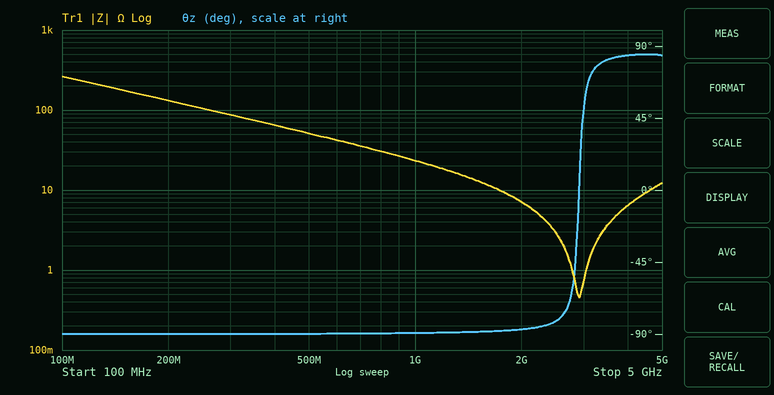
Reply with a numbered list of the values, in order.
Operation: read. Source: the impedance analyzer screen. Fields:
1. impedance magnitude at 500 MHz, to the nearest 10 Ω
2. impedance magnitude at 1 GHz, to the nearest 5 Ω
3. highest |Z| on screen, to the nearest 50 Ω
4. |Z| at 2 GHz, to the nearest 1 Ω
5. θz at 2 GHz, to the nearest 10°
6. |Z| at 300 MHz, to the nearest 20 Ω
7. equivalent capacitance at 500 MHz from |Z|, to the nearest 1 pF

1. 50 Ω
2. 25 Ω
3. 250 Ω
4. 7 Ω
5. -90°
6. 80 Ω
7. 6 pF
